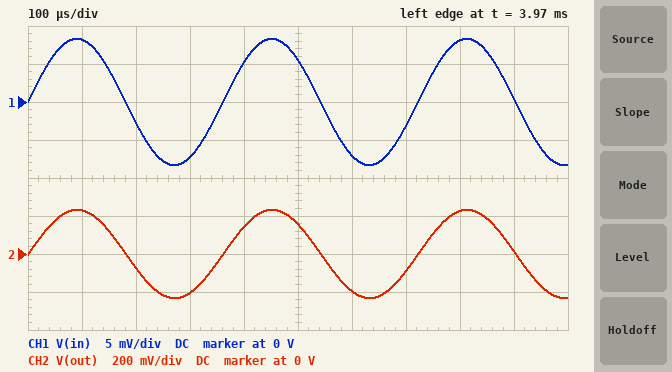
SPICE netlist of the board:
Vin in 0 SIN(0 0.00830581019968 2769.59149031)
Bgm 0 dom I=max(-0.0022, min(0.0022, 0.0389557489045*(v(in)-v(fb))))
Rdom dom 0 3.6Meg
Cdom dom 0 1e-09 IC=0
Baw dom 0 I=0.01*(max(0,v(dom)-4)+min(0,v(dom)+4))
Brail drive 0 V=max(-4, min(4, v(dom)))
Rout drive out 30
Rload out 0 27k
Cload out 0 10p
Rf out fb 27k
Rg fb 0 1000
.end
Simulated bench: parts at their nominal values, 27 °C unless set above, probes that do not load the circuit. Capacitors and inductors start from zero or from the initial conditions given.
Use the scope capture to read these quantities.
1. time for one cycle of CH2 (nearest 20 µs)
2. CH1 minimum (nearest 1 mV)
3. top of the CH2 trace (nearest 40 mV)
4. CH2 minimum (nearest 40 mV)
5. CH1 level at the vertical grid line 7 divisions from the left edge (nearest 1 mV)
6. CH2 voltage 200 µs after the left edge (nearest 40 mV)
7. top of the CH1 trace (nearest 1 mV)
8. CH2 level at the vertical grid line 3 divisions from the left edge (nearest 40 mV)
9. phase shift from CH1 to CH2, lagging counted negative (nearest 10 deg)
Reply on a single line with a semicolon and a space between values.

360 µs; -8 mV; 240 mV; -240 mV; -3 mV; -80 mV; 8 mV; -200 mV; 0 deg
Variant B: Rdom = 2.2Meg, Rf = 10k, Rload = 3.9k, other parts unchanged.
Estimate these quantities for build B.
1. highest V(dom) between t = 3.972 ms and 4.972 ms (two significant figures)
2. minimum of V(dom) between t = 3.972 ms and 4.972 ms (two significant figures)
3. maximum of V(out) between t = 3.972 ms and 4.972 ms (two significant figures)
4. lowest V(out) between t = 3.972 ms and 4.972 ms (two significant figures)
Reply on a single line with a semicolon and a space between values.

92 mV; -92 mV; 91 mV; -91 mV
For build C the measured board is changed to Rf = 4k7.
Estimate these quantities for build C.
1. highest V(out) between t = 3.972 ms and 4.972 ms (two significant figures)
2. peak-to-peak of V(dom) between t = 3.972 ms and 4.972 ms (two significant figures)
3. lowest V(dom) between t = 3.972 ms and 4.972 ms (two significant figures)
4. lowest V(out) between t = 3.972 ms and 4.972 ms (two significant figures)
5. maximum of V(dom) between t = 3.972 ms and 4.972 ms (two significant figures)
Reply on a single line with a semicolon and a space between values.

47 mV; 95 mV; -48 mV; -47 mV; 48 mV
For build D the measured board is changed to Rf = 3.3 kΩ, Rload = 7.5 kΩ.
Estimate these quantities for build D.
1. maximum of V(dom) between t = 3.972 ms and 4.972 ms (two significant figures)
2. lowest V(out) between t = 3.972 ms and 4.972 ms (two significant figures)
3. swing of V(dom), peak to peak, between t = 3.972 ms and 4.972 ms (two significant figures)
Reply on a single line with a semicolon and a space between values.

36 mV; -36 mV; 72 mV
